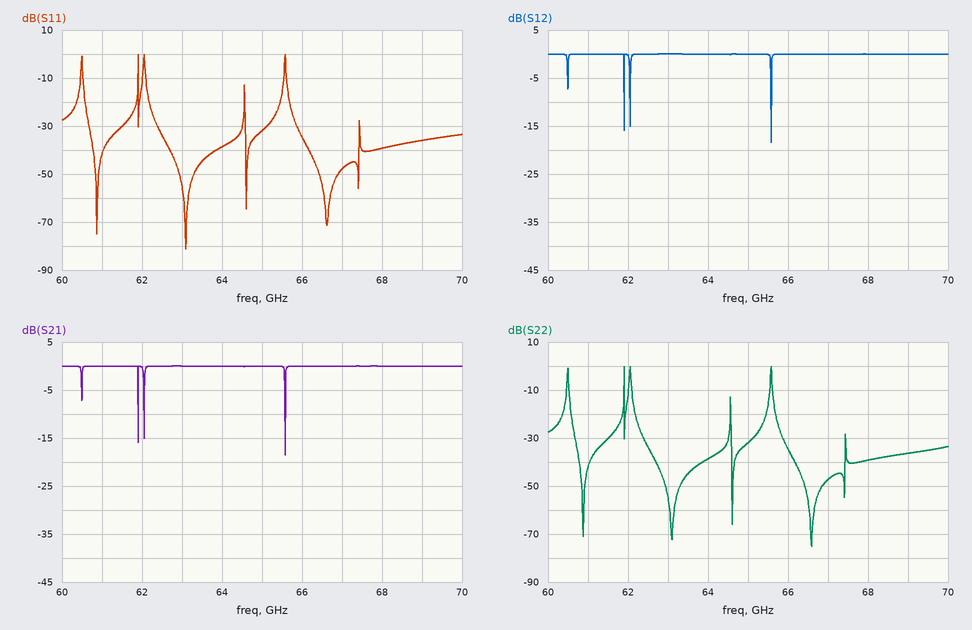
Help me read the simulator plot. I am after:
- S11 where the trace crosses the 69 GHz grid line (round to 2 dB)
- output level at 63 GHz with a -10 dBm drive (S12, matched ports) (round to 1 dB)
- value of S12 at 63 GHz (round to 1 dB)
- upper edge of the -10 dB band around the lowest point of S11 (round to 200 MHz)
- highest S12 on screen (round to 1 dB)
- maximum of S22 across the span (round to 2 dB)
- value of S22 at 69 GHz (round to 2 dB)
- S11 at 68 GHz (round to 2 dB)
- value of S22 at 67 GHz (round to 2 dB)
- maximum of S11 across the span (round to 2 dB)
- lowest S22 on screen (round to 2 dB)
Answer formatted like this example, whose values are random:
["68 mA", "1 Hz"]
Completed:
["-36 dB", "-10 dBm", "0 dB", "65.6 GHz", "0 dB", "0 dB", "-36 dB", "-40 dB", "-48 dB", "0 dB", "-76 dB"]
